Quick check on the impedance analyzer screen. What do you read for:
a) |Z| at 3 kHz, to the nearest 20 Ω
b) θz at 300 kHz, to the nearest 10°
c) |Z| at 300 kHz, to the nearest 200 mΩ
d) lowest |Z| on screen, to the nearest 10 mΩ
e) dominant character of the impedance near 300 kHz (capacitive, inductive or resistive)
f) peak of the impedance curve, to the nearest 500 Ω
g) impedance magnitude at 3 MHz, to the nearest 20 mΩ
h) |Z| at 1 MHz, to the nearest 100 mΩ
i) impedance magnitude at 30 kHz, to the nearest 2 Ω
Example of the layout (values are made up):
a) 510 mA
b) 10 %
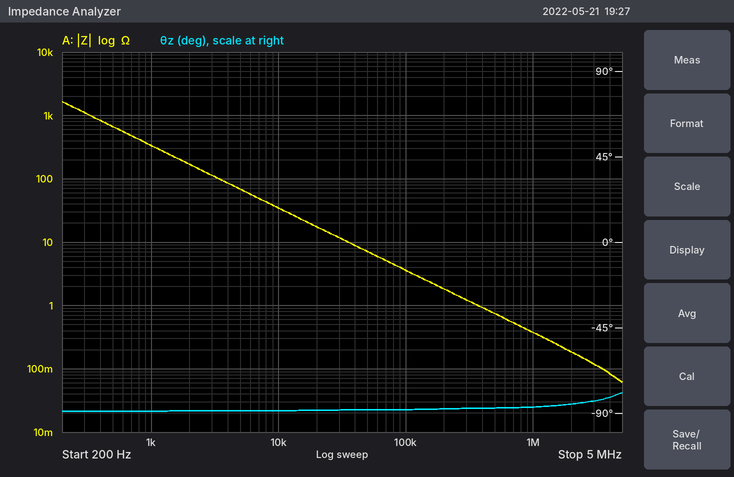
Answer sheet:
a) 120 Ω
b) -90°
c) 1.2 Ω
d) 60 mΩ
e) capacitive
f) 1.5 kΩ
g) 120 mΩ
h) 400 mΩ
i) 12 Ω
